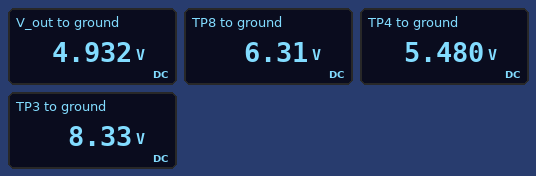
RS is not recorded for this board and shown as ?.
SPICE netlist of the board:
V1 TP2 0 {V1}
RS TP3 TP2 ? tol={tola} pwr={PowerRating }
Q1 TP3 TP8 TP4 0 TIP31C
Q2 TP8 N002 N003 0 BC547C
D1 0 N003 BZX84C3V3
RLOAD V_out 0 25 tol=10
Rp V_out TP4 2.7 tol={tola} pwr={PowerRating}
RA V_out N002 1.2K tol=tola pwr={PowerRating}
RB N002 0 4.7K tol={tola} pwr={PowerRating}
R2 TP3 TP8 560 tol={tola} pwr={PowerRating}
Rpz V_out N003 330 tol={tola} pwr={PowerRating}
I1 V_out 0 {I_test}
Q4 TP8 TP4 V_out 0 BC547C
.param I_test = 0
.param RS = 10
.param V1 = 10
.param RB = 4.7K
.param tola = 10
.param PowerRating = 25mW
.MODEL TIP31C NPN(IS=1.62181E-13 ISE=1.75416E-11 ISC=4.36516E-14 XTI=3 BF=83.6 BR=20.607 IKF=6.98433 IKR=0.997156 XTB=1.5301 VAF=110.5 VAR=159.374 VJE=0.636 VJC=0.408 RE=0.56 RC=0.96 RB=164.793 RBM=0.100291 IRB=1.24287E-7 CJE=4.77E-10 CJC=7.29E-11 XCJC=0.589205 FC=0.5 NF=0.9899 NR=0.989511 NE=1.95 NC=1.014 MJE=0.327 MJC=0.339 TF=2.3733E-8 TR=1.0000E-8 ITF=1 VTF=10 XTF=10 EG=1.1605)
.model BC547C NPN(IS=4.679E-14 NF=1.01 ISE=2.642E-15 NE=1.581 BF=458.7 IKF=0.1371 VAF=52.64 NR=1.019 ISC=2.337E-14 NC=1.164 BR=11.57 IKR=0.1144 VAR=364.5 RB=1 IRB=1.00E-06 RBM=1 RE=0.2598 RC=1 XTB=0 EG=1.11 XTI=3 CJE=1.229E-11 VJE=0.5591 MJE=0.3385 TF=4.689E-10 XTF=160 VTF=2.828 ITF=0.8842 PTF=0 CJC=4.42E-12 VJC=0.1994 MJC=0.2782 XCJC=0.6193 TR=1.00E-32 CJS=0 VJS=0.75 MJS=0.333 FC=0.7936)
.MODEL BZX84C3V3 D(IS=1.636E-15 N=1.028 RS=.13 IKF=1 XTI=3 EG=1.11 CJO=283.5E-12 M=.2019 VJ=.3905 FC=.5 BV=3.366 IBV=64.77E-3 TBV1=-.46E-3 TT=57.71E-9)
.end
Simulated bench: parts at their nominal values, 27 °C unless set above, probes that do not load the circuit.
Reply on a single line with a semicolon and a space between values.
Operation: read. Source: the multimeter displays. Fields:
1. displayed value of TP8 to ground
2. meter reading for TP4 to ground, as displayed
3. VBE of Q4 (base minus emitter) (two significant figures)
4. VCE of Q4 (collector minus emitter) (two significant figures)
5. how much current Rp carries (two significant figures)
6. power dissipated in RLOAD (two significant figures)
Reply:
6.31 V; 5.480 V; 550 mV; 1.4 V; 200 mA; 970 mW
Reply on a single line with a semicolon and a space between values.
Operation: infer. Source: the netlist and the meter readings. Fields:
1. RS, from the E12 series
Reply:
8.2 Ω
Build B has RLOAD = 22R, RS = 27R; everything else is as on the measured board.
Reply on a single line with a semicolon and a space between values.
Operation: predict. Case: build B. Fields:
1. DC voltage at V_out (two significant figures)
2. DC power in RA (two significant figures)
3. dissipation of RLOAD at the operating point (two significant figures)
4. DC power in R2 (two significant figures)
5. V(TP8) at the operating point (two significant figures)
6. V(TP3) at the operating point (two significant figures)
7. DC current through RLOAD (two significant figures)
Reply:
3.4 V; 410 µW; 540 mW; 2.1 mW; 4.7 V; 5.7 V; 160 mA
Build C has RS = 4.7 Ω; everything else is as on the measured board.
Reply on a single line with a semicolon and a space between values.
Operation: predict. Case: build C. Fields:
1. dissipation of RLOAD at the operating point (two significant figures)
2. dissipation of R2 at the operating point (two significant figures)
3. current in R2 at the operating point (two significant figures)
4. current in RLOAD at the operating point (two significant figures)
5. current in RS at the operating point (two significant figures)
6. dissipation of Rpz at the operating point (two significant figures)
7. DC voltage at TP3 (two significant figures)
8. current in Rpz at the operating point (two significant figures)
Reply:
990 mW; 13 mW; 4.8 mA; 200 mA; 210 mA; 8.3 mW; 9.0 V; 5.0 mA
